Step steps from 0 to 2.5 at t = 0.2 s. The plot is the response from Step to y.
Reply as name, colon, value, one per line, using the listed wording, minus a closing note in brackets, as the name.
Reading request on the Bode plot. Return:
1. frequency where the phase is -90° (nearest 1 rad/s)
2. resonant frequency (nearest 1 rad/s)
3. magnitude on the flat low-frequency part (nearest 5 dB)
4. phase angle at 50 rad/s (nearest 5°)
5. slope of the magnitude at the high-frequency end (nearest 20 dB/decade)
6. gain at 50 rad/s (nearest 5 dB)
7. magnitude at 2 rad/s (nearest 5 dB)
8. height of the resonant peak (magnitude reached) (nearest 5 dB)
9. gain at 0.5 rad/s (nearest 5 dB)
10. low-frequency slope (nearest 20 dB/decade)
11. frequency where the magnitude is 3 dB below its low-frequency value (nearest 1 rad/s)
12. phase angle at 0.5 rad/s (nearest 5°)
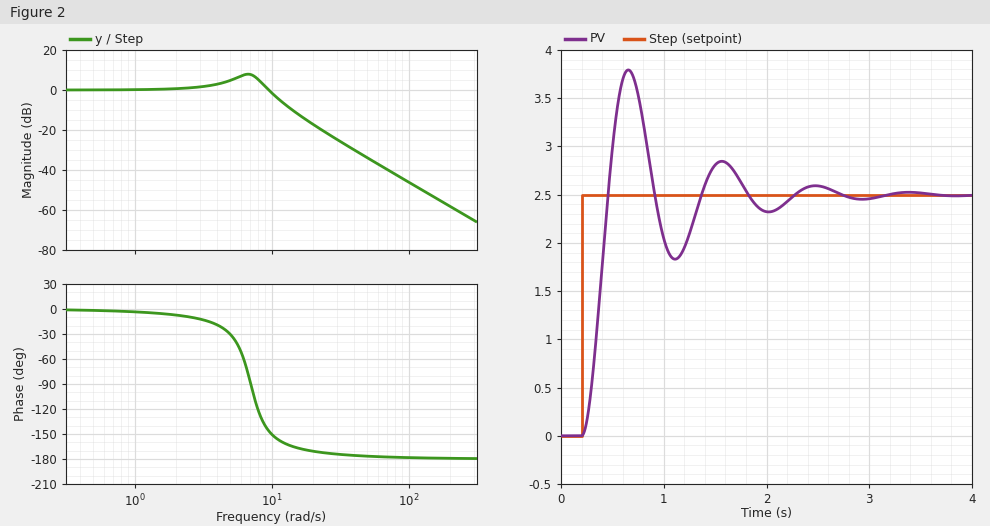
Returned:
frequency where the phase is -90°: 7 rad/s
resonant frequency: 7 rad/s
magnitude on the flat low-frequency part: 0 dB
phase angle at 50 rad/s: -175°
slope of the magnitude at the high-frequency end: -40 dB/decade
gain at 50 rad/s: -35 dB
magnitude at 2 rad/s: 0 dB
height of the resonant peak (magnitude reached): 10 dB
gain at 0.5 rad/s: 0 dB
low-frequency slope: 0 dB/decade
frequency where the magnitude is 3 dB below its low-frequency value: 11 rad/s
phase angle at 0.5 rad/s: 0°
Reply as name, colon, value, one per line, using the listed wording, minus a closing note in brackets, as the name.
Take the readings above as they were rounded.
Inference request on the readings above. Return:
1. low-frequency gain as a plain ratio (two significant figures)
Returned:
low-frequency gain as a plain ratio: 1.0
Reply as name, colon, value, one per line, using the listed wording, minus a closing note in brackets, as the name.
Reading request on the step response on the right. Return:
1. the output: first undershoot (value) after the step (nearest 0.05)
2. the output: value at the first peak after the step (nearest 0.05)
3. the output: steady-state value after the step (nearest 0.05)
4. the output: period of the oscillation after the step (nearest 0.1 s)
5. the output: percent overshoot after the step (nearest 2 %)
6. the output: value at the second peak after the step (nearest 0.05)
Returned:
the output: first undershoot (value) after the step: 1.85
the output: value at the first peak after the step: 3.80
the output: steady-state value after the step: 2.50
the output: period of the oscillation after the step: 0.9 s
the output: percent overshoot after the step: 52 %
the output: value at the second peak after the step: 2.85
